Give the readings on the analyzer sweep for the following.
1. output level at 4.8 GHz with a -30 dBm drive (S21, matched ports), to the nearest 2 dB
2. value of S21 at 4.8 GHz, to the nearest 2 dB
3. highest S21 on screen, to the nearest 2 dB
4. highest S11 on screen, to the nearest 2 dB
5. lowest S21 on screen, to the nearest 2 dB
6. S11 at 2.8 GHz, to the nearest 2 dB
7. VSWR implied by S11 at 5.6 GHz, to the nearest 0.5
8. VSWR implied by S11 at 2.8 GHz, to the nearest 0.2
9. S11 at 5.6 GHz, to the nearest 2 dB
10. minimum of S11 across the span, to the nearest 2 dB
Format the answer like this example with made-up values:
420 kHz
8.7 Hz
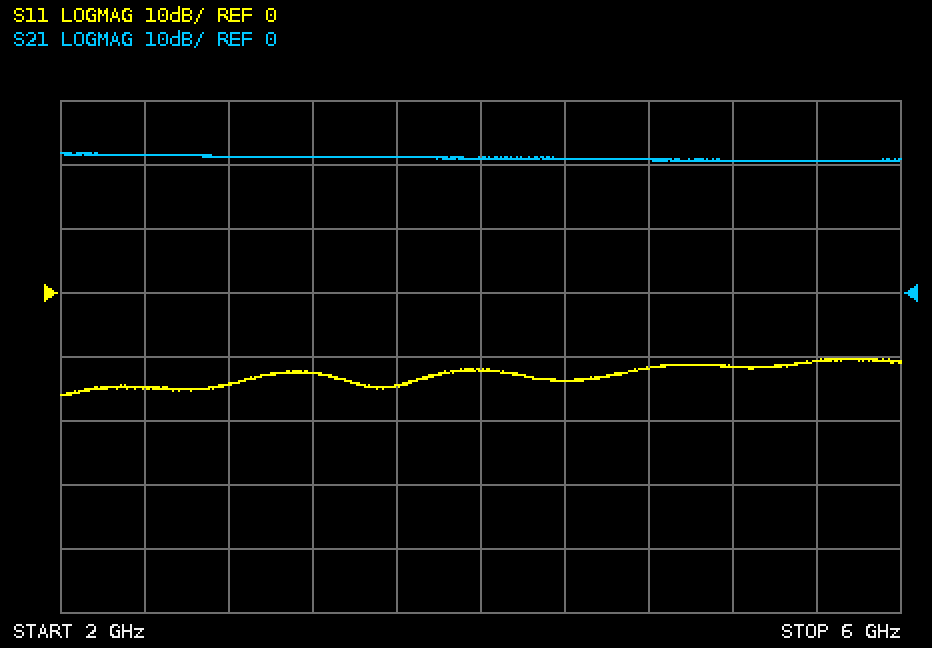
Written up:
-10 dBm
20 dB
22 dB
-10 dB
20 dB
-14 dB
2.0
1.4
-10 dB
-16 dB
